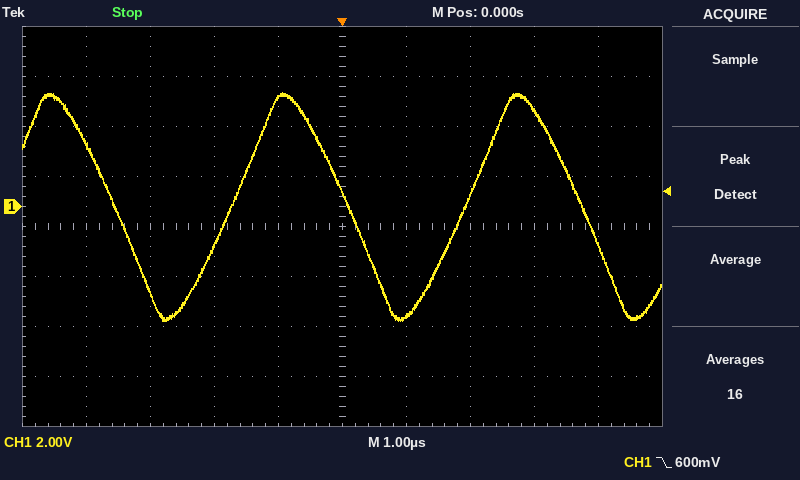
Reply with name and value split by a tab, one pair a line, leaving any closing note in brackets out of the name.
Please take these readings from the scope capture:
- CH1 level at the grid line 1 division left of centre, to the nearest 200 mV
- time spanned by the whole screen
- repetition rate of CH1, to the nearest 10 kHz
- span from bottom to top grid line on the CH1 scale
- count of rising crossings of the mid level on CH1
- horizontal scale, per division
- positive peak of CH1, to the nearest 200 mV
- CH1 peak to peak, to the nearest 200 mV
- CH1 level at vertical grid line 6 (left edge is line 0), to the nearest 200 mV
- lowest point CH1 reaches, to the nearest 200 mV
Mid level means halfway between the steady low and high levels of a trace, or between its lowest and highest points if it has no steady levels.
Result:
CH1 level at the grid line 1 division left of centre, to the nearest 200 mV	4.4 V
time spanned by the whole screen	10 µs
repetition rate of CH1, to the nearest 10 kHz	270 kHz
span from bottom to top grid line on the CH1 scale	16 V
count of rising crossings of the mid level on CH1	2
horizontal scale, per division	1 µs
positive peak of CH1, to the nearest 200 mV	4.6 V
CH1 peak to peak, to the nearest 200 mV	9.2 V
CH1 level at vertical grid line 6 (left edge is line 0), to the nearest 200 mV	-4.4 V
lowest point CH1 reaches, to the nearest 200 mV	-4.6 V
